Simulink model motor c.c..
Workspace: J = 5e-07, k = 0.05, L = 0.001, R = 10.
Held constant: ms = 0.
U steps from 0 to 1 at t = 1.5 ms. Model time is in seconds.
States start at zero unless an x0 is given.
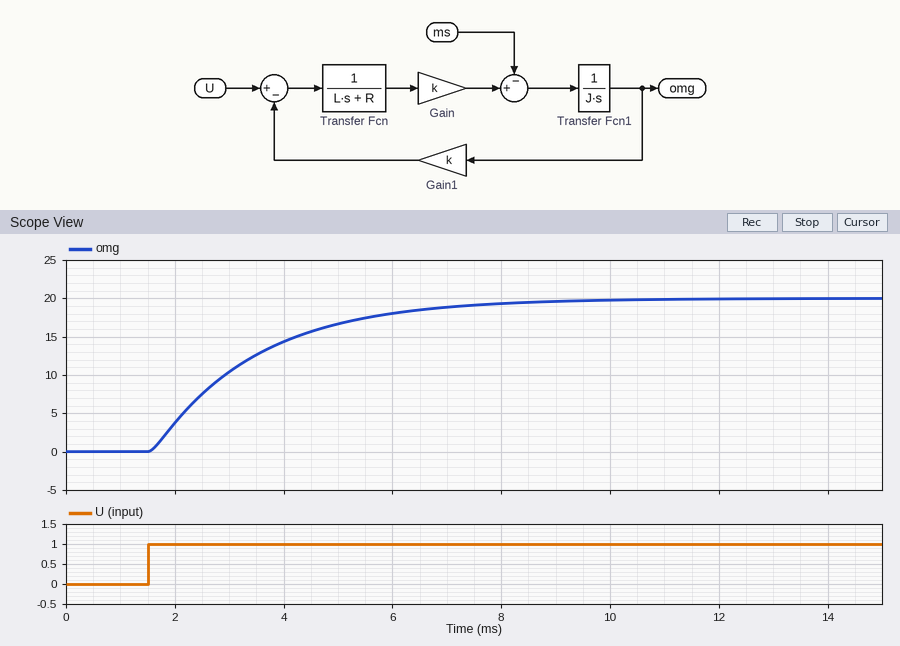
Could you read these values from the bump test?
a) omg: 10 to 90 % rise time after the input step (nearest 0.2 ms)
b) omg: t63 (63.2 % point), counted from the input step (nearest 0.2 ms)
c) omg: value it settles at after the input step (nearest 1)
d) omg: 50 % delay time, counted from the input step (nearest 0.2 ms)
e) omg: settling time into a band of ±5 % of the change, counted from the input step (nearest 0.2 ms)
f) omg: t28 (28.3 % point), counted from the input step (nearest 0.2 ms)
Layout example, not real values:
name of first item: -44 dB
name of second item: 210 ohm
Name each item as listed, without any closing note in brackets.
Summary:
omg: 10 to 90 % rise time after the input step: 4.2 ms
omg: t63 (63.2 % point), counted from the input step: 2.0 ms
omg: value it settles at after the input step: 20
omg: 50 % delay time, counted from the input step: 1.4 ms
omg: settling time into a band of ±5 % of the change, counted from the input step: 5.8 ms
omg: t28 (28.3 % point), counted from the input step: 0.8 ms
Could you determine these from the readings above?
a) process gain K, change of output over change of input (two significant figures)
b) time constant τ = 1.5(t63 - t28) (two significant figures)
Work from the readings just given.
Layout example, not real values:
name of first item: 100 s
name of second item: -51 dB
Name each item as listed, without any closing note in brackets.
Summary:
process gain K, change of output over change of input: 20
time constant τ = 1.5(t63 - t28): 1.8 ms
